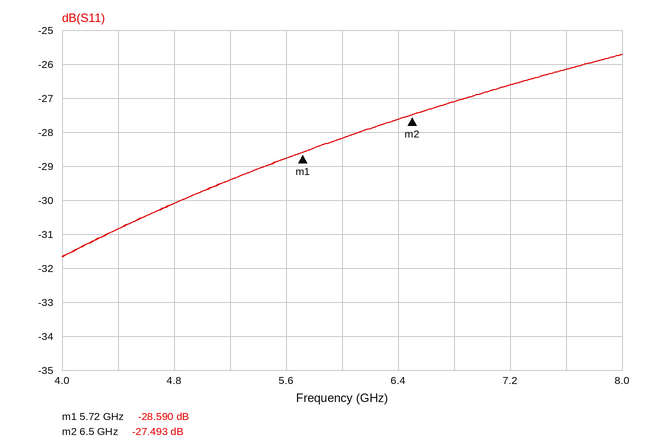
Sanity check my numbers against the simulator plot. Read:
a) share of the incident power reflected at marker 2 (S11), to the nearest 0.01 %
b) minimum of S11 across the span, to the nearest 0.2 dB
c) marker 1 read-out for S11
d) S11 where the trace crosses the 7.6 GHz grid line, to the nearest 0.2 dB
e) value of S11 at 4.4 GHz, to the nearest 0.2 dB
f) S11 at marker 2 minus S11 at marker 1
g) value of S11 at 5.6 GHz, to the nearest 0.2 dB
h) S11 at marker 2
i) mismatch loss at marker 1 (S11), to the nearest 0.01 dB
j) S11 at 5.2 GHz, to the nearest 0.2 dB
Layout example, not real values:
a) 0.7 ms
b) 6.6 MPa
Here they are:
a) 0.18 %
b) -31.6 dB
c) -28.590 dB
d) -26.2 dB
e) -30.8 dB
f) 1.097 dB
g) -28.8 dB
h) -27.493 dB
i) 0.01 dB
j) -29.4 dB
